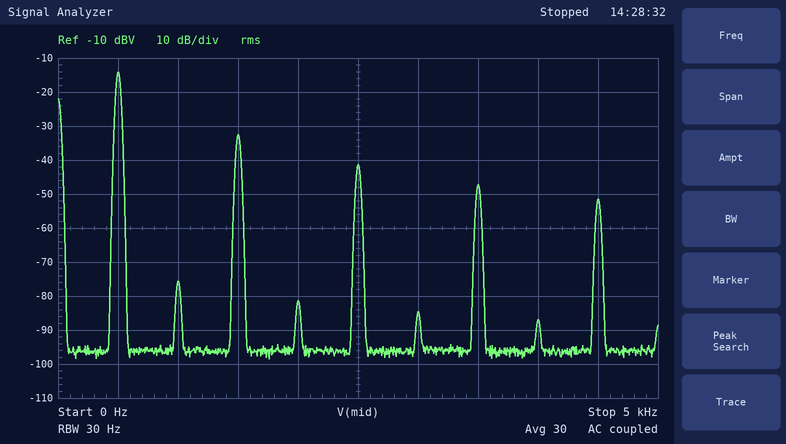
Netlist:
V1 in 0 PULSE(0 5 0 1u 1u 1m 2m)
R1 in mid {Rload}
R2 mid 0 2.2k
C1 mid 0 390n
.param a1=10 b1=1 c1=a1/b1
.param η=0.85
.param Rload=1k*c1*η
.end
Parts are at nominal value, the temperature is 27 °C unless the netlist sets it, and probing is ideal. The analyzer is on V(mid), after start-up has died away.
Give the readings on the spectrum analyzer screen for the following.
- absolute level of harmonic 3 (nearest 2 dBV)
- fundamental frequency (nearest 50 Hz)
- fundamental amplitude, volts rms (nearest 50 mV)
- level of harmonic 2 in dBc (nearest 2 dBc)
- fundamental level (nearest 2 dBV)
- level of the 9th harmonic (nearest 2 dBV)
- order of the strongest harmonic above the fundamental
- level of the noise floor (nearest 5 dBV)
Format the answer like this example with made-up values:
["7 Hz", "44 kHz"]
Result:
["-32 dBV", "500 Hz", "200 mV", "-62 dBc", "-14 dBV", "-52 dBV", "3", "-95 dBV"]
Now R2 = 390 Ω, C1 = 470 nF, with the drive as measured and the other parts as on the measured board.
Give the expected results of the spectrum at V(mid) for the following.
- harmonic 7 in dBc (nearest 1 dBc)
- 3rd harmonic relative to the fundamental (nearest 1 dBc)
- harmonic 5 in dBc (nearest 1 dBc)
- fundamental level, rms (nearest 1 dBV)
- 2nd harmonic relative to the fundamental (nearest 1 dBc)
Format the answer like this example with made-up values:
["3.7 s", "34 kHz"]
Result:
["-28 dBc", "-14 dBc", "-22 dBc", "-21 dBV", "-58 dBc"]
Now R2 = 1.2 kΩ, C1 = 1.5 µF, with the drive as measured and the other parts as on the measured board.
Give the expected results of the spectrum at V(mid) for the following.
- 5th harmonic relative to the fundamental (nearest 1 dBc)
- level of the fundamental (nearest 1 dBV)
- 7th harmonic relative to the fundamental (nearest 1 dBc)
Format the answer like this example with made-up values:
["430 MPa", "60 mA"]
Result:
["-28 dBc", "-25 dBV", "-34 dBc"]
